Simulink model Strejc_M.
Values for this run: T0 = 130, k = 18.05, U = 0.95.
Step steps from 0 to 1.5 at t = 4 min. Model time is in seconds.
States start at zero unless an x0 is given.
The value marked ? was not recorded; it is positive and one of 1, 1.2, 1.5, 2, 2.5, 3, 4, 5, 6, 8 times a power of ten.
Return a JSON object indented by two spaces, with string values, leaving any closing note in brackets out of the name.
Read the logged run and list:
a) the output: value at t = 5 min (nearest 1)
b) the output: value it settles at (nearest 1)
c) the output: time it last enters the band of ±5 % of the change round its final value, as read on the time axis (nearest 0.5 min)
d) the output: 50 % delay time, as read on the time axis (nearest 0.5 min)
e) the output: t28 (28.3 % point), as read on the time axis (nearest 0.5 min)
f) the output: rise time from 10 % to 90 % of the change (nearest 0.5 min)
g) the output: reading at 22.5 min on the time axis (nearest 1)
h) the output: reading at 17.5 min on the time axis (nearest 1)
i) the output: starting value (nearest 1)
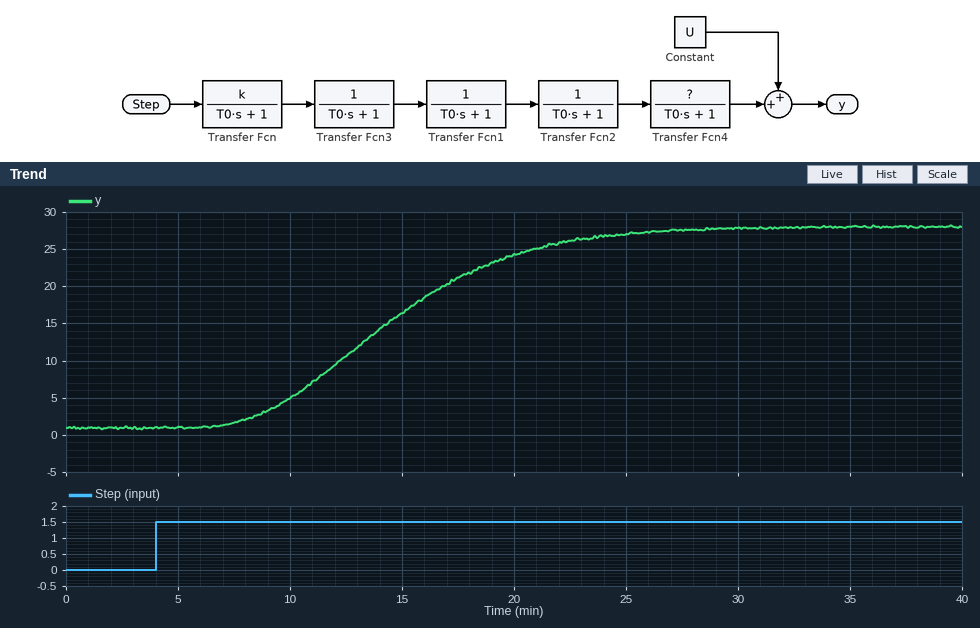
{
  "the output: value at t = 5 min": "1",
  "the output: value it settles at": "28",
  "the output: time it last enters the band of ±5 % of the change round its final value, as read on the time axis": "24.0 min",
  "the output: 50 % delay time, as read on the time axis": "14.0 min",
  "the output: t28 (28.3 % point), as read on the time axis": "11.5 min",
  "the output: rise time from 10 % to 90 % of the change": "12.0 min",
  "the output: reading at 22.5 min on the time axis": "26",
  "the output: reading at 17.5 min on the time axis": "21",
  "the output: starting value": "1"
}
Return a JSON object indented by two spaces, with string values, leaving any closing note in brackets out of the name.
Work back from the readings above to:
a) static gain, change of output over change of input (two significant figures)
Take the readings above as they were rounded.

{
  "static gain, change of output over change of input": "18"
}
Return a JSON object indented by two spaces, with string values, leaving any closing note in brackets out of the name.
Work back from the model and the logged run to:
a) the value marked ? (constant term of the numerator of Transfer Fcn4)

{
  "the value marked ?": "1"
}
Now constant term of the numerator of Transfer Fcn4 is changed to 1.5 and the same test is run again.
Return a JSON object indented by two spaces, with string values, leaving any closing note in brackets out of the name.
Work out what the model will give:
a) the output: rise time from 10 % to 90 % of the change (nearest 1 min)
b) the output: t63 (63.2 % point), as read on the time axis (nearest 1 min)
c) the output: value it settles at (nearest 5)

{
  "the output: rise time from 10 % to 90 % of the change": "12 min",
  "the output: t63 (63.2 % point), as read on the time axis": "16 min",
  "the output: value it settles at": "40"
}
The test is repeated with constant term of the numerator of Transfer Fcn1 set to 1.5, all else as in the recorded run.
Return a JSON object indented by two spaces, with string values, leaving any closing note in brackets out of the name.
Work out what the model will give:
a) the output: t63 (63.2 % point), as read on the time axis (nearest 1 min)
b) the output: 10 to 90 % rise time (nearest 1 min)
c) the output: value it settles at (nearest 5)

{
  "the output: t63 (63.2 % point), as read on the time axis": "16 min",
  "the output: 10 to 90 % rise time": "12 min",
  "the output: value it settles at": "40"
}
